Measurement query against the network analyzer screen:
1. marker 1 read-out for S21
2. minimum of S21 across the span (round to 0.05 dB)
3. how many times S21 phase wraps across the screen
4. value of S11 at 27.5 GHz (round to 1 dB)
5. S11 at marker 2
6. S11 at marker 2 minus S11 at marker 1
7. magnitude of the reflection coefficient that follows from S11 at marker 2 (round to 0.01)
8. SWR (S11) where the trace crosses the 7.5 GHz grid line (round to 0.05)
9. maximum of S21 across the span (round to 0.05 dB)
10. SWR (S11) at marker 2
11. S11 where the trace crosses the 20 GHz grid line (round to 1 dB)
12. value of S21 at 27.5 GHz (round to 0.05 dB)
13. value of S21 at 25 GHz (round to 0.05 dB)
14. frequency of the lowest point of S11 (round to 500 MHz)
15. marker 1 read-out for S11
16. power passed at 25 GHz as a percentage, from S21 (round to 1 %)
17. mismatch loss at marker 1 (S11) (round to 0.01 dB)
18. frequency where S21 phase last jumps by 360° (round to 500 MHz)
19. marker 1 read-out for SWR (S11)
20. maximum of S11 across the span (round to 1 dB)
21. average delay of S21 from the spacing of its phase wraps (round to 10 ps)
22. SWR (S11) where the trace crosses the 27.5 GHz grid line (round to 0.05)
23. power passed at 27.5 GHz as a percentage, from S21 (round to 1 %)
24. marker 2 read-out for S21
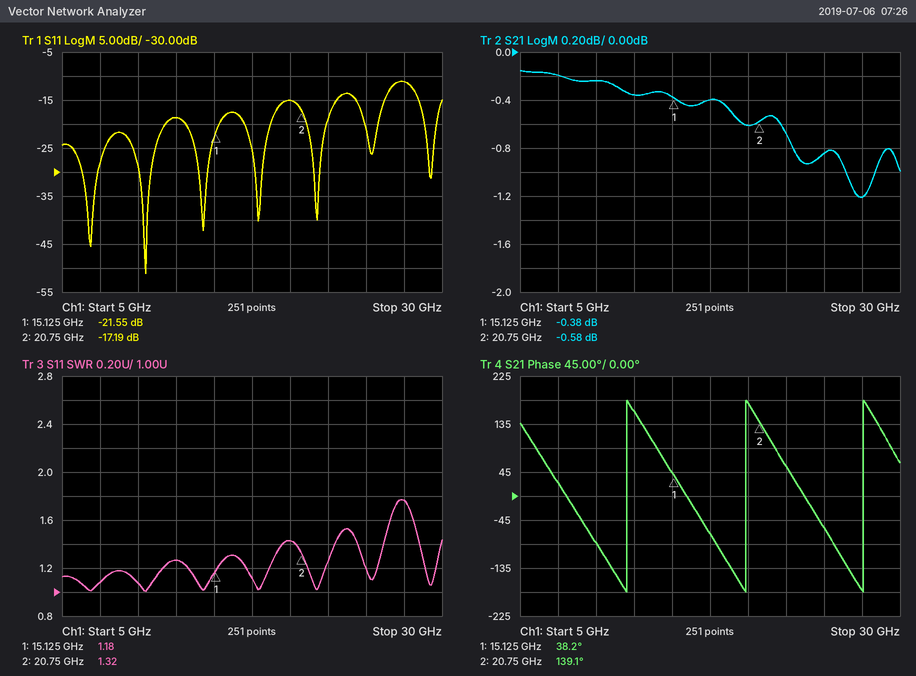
-0.38 dB
-1.20 dB
3
-11 dB
-17.19 dB
4.36 dB
0.14
1.10
-0.15 dB
1.32
-15 dB
-1.20 dB
-0.85 dB
10.5 GHz
-21.55 dB
82 %
0.03 dB
27.5 GHz
1.18
-11 dB
130 ps
1.75
76 %
-0.58 dB
